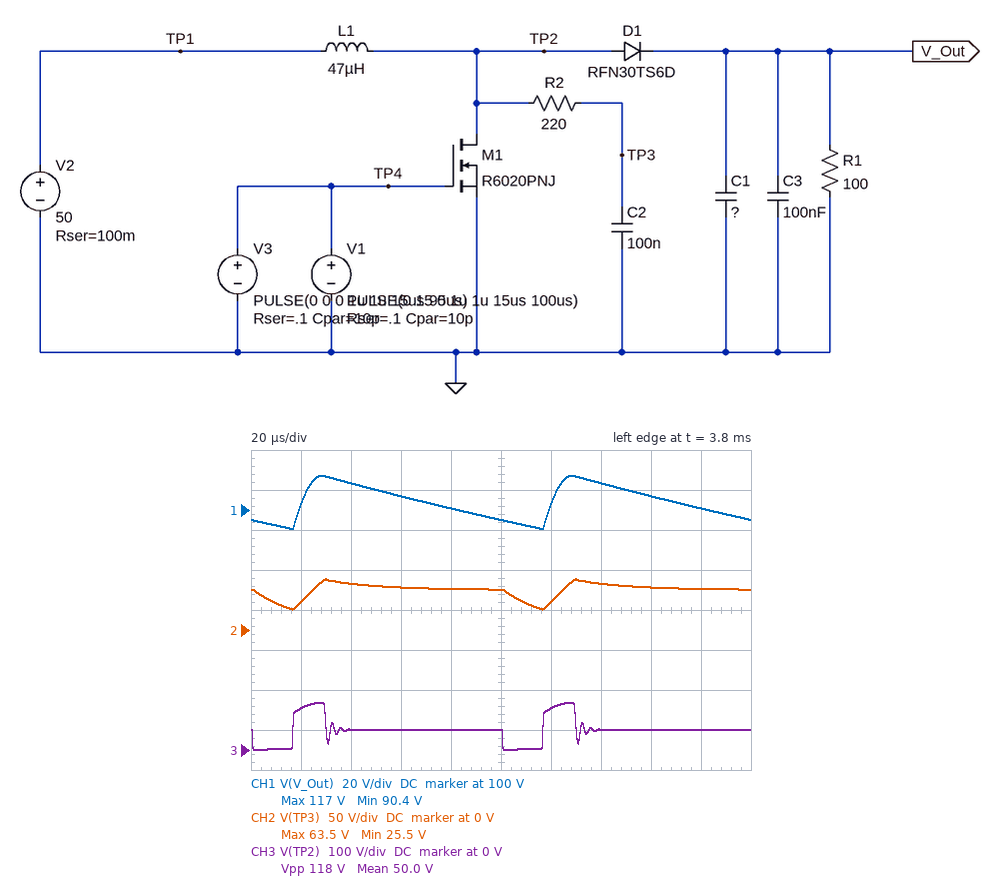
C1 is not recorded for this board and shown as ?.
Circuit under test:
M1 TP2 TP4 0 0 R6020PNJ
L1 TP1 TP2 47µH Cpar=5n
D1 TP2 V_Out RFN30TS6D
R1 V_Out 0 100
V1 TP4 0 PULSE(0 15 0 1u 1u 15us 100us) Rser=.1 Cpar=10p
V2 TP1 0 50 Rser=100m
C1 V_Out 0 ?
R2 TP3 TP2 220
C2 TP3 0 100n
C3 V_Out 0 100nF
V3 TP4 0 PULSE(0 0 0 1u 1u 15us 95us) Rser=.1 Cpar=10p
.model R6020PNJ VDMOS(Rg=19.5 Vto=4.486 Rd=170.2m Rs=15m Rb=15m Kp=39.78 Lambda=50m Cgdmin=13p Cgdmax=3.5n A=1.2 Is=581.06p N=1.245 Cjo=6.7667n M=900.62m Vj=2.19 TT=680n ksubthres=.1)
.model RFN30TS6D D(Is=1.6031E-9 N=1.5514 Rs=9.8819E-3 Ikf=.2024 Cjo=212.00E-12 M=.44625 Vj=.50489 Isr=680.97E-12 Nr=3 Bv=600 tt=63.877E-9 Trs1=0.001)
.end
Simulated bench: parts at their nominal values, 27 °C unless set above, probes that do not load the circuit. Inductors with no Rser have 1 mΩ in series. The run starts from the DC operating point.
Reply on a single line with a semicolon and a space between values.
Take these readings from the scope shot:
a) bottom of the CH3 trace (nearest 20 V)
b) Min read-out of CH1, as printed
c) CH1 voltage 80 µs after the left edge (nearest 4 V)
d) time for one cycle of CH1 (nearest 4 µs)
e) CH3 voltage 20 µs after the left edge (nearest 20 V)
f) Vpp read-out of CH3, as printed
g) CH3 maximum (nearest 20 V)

0 V; 90.4 V; 100 V; 100 µs; 100 V; 118 V; 120 V
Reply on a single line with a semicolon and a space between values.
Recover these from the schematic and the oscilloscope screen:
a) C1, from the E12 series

3.3 µF
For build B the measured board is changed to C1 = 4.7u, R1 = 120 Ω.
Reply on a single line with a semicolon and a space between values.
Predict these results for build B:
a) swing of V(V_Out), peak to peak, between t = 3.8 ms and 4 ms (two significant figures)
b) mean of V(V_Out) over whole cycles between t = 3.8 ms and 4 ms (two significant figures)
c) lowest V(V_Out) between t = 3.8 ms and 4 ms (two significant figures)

17 V; 110 V; 100 V
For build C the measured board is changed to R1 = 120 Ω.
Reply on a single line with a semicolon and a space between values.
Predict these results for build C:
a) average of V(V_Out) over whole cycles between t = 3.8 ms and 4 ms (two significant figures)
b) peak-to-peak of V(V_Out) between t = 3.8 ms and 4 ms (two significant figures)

110 V; 24 V
